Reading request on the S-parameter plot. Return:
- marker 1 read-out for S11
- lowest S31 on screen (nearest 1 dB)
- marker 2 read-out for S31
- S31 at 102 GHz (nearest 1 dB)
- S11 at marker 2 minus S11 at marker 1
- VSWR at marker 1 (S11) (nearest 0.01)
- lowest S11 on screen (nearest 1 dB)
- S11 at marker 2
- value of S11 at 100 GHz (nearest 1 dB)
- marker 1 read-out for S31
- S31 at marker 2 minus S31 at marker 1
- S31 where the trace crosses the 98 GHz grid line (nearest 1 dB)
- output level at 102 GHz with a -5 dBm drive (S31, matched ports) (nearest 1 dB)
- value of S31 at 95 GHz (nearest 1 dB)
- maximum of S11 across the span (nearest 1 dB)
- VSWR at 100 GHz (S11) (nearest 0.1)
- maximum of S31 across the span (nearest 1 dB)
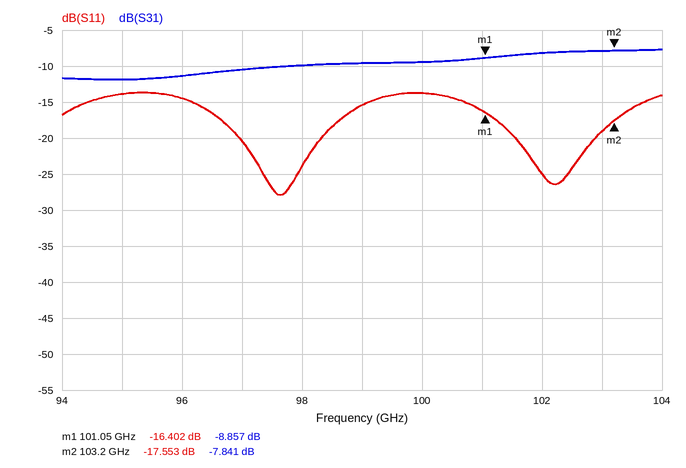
-16.402 dB
-12 dB
-7.841 dB
-8 dB
-1.151 dB
1.36
-28 dB
-17.553 dB
-14 dB
-8.857 dB
1.016 dB
-10 dB
-13 dBm
-12 dB
-14 dB
1.5
-8 dB
